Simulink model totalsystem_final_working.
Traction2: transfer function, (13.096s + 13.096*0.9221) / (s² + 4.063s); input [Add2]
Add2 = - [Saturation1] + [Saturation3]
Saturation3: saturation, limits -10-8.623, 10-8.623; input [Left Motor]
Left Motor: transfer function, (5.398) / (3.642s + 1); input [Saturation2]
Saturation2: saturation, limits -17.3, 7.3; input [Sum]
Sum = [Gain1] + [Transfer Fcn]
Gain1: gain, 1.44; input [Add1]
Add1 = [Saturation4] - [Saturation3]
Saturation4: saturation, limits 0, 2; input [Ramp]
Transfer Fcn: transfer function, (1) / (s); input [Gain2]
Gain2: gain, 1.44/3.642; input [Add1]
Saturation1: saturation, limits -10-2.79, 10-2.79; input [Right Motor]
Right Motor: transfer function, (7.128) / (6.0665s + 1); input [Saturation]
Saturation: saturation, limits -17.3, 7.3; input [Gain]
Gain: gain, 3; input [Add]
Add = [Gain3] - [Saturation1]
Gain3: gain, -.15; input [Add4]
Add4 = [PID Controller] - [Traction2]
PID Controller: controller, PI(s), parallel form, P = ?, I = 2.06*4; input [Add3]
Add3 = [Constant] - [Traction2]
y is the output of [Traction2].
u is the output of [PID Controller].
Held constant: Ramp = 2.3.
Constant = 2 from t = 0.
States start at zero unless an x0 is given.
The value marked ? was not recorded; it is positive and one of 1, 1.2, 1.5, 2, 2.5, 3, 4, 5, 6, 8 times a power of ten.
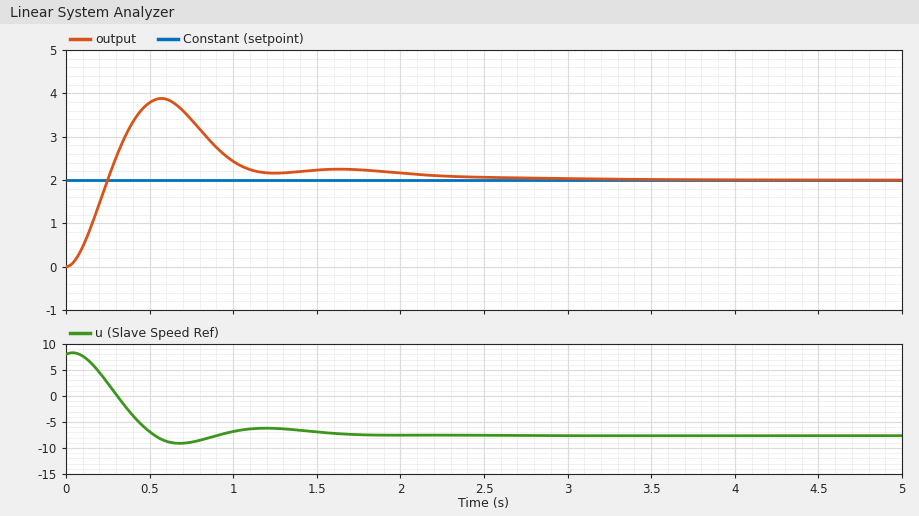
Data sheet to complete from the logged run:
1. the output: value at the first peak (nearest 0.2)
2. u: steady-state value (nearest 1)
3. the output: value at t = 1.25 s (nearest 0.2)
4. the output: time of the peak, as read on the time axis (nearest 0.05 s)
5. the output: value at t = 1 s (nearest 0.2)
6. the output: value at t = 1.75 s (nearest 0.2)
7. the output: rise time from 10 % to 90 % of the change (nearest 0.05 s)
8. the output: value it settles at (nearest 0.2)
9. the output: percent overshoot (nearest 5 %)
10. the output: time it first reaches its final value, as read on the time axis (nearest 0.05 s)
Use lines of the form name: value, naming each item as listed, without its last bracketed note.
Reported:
the output: value at the first peak: 3.8
u: steady-state value: -8
the output: value at t = 1.25 s: 2.2
the output: time of the peak, as read on the time axis: 0.55 s
the output: value at t = 1 s: 2.4
the output: value at t = 1.75 s: 2.2
the output: rise time from 10 % to 90 % of the change: 0.15 s
the output: value it settles at: 2.0
the output: percent overshoot: 95 %
the output: time it first reaches its final value, as read on the time axis: 0.25 s
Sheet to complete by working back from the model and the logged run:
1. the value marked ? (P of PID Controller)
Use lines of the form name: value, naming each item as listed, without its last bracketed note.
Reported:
the value marked ?: 4
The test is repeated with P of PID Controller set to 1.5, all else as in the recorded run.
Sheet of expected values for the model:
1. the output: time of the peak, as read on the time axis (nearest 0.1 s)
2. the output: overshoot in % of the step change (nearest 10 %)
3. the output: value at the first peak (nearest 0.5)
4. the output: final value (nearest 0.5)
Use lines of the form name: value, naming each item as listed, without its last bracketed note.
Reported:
the output: time of the peak, as read on the time axis: 0.7 s
the output: overshoot in % of the step change: 120 %
the output: value at the first peak: 4.5
the output: final value: 2.0
